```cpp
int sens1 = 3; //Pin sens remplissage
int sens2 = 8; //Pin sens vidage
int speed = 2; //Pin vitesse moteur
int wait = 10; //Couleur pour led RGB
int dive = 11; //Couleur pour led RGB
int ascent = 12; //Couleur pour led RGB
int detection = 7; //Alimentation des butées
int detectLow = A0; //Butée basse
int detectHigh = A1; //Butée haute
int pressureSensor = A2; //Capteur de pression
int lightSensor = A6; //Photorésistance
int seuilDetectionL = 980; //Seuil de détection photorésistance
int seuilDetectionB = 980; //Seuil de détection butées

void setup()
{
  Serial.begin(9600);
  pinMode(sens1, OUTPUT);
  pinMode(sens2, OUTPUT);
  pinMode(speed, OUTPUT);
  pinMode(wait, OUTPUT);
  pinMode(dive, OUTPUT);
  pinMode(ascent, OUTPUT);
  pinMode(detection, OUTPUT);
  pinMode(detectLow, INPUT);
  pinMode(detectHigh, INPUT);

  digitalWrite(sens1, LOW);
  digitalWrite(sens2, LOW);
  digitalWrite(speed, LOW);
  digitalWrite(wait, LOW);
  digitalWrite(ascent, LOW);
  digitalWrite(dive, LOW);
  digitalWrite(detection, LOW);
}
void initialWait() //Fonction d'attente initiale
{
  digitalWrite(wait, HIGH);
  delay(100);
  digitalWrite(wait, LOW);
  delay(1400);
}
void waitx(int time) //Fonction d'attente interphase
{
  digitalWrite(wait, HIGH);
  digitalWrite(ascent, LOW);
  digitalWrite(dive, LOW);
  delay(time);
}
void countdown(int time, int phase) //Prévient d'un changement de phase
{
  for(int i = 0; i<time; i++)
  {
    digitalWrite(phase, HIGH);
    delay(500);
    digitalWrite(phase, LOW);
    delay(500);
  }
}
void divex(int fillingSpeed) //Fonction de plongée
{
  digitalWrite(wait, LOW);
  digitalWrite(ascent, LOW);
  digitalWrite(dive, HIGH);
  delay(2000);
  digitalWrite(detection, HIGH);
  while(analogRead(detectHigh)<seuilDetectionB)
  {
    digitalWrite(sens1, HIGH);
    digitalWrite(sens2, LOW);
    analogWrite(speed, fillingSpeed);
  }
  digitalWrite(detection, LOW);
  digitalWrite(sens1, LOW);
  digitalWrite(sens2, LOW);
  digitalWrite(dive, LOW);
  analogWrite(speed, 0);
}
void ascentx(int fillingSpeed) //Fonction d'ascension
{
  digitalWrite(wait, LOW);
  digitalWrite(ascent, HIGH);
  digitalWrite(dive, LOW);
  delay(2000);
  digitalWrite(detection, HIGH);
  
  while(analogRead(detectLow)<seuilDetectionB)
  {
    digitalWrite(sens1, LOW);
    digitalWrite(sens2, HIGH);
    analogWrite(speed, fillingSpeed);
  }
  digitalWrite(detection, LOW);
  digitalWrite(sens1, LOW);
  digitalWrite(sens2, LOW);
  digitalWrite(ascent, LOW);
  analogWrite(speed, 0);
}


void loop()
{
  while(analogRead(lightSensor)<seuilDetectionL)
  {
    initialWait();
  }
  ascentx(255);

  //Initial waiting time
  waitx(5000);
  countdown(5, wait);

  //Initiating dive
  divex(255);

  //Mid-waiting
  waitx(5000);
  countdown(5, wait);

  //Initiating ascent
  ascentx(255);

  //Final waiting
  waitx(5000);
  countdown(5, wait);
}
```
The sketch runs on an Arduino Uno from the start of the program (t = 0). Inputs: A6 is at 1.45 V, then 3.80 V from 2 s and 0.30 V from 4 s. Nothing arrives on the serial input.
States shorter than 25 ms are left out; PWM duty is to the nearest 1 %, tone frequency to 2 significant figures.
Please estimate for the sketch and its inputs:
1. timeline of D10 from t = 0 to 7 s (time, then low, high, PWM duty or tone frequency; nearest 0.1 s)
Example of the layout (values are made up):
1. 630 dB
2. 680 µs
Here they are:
1. 0 s high; 0.1 s low; 1.5 s high; 1.6 s low; 3 s high; 3.1 s low; 4.5 s high; 4.6 s low; 6 s high; 6.1 s low
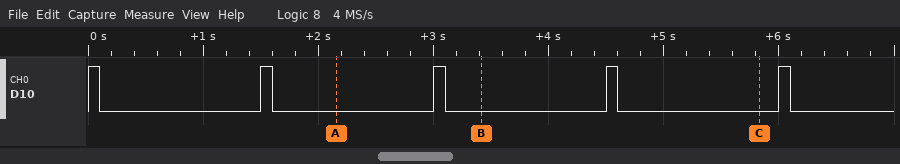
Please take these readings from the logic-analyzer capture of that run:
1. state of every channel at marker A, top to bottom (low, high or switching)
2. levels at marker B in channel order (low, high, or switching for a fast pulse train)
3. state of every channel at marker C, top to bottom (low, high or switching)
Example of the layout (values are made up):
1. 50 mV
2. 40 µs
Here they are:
1. D10 low
2. D10 low
3. D10 low
